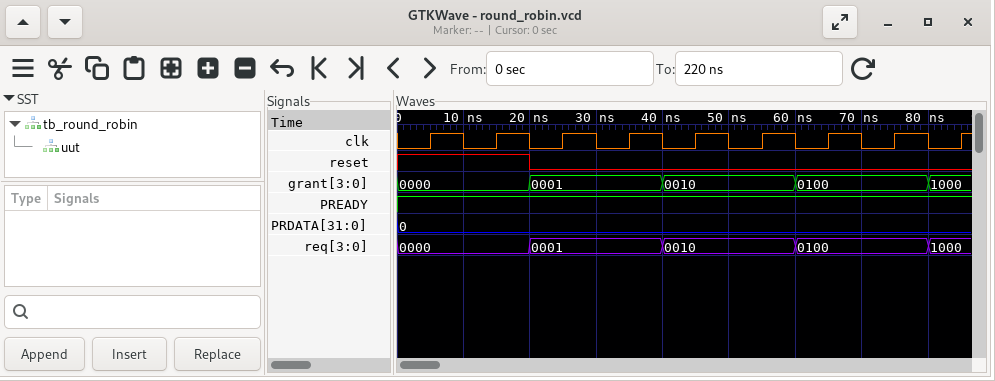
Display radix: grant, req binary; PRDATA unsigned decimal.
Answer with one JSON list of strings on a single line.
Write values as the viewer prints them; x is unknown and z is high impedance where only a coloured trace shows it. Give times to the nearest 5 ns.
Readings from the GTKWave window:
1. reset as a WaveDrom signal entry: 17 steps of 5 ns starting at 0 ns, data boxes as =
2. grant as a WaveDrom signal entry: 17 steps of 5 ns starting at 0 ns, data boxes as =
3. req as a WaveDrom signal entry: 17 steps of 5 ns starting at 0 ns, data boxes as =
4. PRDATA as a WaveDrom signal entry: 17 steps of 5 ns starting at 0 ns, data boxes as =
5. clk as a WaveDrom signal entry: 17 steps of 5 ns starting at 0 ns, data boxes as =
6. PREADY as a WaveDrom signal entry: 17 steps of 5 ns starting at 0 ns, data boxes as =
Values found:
["{name: 'reset', wave: '1...0............'}", "{name: 'grant', wave: '=...=...=...=...=', data: '0000 0001 0010 0100 1000'}", "{name: 'req', wave: '=...=...=...=...=', data: '0000 0001 0010 0100 1000'}", "{name: 'PRDATA', wave: '=................', data: '0'}", "{name: 'clk', wave: '01010101010101010'}", "{name: 'PREADY', wave: '1................'}"]
